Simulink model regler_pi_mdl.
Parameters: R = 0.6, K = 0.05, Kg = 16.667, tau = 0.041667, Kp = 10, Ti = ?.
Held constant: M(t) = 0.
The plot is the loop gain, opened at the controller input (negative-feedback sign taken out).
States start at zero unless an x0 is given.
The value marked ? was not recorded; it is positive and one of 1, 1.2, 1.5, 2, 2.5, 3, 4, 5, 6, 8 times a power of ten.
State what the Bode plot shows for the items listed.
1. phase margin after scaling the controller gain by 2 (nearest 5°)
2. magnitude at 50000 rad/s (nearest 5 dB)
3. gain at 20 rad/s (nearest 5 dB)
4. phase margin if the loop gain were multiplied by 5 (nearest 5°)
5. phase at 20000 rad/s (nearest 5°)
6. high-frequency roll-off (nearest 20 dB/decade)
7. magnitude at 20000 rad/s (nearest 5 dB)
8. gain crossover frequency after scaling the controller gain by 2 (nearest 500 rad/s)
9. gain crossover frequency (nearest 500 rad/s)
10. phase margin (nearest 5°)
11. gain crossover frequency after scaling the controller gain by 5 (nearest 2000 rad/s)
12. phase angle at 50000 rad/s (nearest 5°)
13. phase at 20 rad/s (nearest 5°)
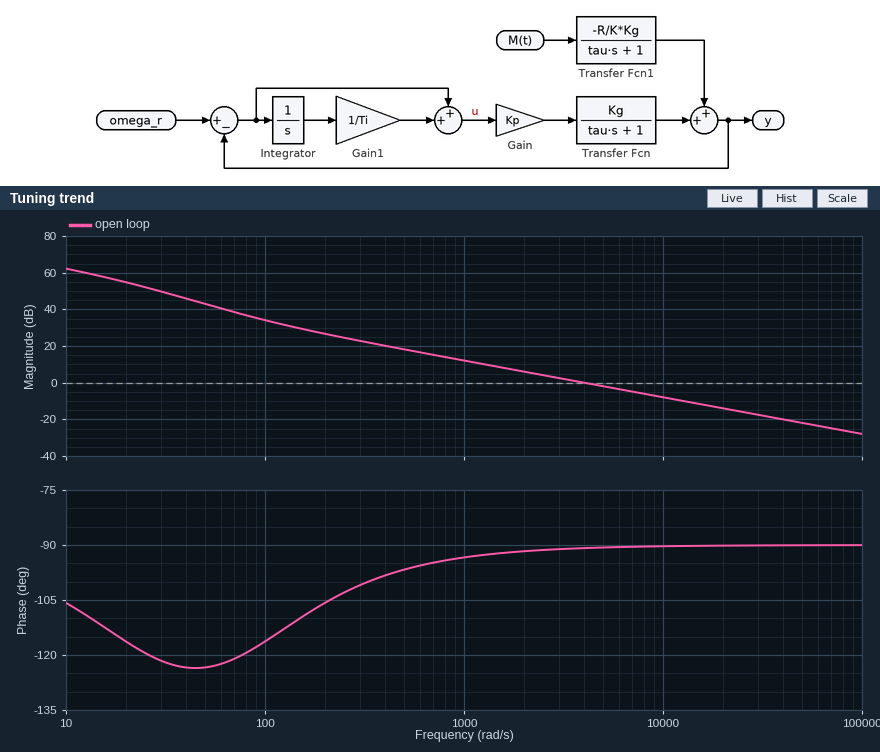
90°
-20 dB
55 dB
90°
-90°
-20 dB/decade
-15 dB
8000 rad/s
4000 rad/s
90°
20000 rad/s
-90°
-115°
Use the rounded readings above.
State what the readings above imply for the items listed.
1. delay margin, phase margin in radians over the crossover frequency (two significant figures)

0.00039 s
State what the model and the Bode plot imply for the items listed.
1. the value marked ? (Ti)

0.012
